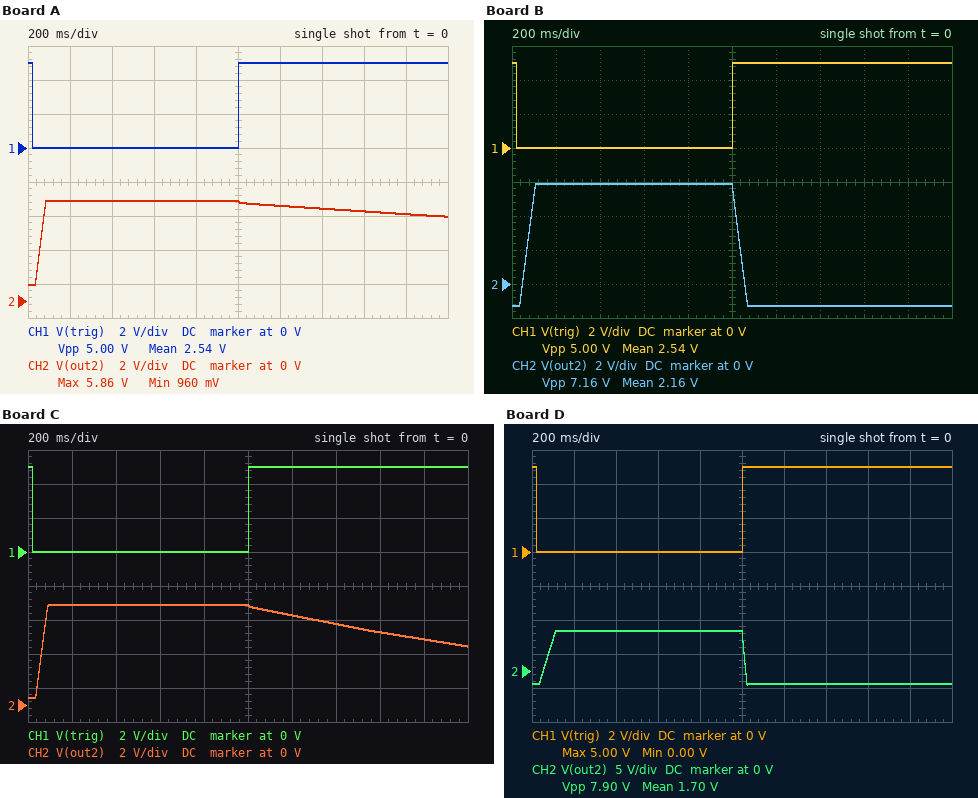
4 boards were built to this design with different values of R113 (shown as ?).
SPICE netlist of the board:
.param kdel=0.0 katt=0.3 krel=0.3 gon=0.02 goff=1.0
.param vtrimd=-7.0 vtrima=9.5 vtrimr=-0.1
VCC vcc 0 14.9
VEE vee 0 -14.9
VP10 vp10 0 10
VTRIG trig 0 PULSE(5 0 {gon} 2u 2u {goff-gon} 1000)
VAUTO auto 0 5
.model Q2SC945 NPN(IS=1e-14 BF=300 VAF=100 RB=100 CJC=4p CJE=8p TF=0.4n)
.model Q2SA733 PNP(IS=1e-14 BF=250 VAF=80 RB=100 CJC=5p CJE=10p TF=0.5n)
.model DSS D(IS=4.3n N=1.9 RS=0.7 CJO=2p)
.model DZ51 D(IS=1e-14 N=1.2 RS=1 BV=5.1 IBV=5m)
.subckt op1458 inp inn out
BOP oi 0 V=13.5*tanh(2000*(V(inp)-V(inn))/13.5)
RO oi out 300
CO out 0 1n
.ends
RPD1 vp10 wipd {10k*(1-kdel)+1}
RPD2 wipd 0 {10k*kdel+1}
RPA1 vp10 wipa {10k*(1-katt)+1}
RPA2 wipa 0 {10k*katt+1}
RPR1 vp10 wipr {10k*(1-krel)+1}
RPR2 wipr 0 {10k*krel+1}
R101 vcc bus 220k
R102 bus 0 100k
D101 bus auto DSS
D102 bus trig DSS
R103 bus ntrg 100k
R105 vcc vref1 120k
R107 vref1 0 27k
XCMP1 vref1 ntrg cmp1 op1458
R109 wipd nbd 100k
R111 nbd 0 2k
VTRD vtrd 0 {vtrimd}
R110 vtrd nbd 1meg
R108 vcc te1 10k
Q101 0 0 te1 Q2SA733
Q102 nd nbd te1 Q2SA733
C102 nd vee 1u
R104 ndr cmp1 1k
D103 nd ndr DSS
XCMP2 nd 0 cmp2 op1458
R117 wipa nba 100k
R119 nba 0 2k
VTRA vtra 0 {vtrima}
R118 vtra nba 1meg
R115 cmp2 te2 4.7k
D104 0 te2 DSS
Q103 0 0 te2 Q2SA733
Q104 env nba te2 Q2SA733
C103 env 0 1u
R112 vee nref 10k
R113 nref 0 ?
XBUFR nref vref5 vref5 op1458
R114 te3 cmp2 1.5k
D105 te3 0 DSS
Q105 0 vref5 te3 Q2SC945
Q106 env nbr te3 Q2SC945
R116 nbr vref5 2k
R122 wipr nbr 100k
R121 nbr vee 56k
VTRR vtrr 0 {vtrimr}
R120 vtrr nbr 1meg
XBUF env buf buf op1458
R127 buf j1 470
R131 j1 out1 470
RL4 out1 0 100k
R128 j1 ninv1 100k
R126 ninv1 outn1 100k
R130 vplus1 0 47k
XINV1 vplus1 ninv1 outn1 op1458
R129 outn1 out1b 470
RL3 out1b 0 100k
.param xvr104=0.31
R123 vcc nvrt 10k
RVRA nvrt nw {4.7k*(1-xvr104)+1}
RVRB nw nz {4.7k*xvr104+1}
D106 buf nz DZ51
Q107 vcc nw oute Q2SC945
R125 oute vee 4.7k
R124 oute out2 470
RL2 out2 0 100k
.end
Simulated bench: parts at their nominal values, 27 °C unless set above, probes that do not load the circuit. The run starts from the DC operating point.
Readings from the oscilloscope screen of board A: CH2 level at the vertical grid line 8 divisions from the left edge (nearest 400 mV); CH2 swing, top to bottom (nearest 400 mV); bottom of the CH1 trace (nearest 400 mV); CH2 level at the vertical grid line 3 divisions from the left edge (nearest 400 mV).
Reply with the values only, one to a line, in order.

5.2 V
4.8 V
0 V
6.0 V
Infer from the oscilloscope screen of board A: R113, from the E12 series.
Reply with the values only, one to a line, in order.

3.9 kΩ
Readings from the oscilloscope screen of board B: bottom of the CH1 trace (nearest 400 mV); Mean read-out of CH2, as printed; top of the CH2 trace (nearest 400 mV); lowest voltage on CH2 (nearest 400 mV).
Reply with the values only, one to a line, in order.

0 V
2.16 V
6.0 V
-1.2 V
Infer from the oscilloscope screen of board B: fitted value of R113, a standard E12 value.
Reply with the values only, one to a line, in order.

8.2 kΩ
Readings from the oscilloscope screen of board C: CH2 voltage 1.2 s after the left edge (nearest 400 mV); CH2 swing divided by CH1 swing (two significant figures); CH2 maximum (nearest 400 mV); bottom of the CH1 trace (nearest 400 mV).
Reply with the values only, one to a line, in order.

5.2 V
1.1
6.0 V
0 V
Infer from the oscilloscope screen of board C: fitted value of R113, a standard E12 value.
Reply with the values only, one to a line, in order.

4.7 kΩ
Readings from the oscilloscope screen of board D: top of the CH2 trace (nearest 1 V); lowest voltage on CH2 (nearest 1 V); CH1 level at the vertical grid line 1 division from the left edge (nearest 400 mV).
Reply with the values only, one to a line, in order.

6 V
-2 V
0 V
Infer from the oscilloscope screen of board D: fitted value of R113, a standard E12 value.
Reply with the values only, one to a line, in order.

10 kΩ
